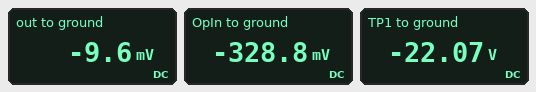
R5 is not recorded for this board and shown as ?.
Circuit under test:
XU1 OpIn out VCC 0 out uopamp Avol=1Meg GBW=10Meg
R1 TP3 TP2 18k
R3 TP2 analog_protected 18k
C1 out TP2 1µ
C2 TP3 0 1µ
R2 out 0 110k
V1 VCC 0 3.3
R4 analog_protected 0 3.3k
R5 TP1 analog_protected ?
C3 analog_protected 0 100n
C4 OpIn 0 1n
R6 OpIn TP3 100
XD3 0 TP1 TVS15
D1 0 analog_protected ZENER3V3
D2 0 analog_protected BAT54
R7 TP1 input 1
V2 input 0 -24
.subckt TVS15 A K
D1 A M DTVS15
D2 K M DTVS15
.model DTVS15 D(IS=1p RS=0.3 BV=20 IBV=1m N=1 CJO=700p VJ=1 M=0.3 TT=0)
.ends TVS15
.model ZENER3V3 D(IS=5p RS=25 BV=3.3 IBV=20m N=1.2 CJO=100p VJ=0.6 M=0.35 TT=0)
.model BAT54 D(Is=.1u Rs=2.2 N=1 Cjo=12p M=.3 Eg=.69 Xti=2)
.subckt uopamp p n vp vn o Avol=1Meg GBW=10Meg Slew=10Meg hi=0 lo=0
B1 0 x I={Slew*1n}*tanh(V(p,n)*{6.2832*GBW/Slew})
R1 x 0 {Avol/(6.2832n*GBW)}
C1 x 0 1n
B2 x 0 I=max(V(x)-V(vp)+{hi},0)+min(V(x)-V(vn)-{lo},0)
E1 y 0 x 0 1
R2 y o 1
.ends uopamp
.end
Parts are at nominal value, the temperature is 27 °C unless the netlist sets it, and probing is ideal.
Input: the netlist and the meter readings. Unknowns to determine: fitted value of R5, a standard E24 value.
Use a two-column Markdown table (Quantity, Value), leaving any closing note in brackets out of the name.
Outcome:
| Quantity | Value |
|---|---|
| fitted value of R5, a standard E24 value | 1.8 kΩ |
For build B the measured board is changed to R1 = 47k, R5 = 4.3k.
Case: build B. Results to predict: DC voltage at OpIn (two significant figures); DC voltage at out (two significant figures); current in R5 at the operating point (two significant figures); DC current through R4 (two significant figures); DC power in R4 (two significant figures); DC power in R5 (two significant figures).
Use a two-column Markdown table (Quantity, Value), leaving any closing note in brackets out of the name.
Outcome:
| Quantity | Value |
|---|---|
| DC voltage at OpIn | -290 mV |
| DC voltage at out | -9.4 mV |
| current in R5 at the operating point | 5.1 mA |
| DC current through R4 | 88 µA |
| DC power in R4 | 26 µW |
| DC power in R5 | 110 mW |
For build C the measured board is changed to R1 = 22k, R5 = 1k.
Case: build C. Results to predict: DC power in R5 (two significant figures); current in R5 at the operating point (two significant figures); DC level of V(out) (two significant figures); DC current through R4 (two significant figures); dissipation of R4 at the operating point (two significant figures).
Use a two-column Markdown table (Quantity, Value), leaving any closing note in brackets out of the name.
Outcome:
| Quantity | Value |
|---|---|
| DC power in R5 | 470 mW |
| current in R5 at the operating point | 22 mA |
| DC level of V(out) | -9.8 mV |
| DC current through R4 | 110 µA |
| dissipation of R4 at the operating point | 40 µW |
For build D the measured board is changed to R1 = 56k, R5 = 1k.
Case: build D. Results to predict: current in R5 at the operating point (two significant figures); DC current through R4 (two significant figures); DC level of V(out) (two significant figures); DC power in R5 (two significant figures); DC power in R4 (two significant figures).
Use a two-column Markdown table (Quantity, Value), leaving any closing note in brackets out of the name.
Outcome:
| Quantity | Value |
|---|---|
| current in R5 at the operating point | 22 mA |
| DC current through R4 | 110 µA |
| DC level of V(out) | -9.8 mV |
| DC power in R5 | 470 mW |
| DC power in R4 | 40 µW |
